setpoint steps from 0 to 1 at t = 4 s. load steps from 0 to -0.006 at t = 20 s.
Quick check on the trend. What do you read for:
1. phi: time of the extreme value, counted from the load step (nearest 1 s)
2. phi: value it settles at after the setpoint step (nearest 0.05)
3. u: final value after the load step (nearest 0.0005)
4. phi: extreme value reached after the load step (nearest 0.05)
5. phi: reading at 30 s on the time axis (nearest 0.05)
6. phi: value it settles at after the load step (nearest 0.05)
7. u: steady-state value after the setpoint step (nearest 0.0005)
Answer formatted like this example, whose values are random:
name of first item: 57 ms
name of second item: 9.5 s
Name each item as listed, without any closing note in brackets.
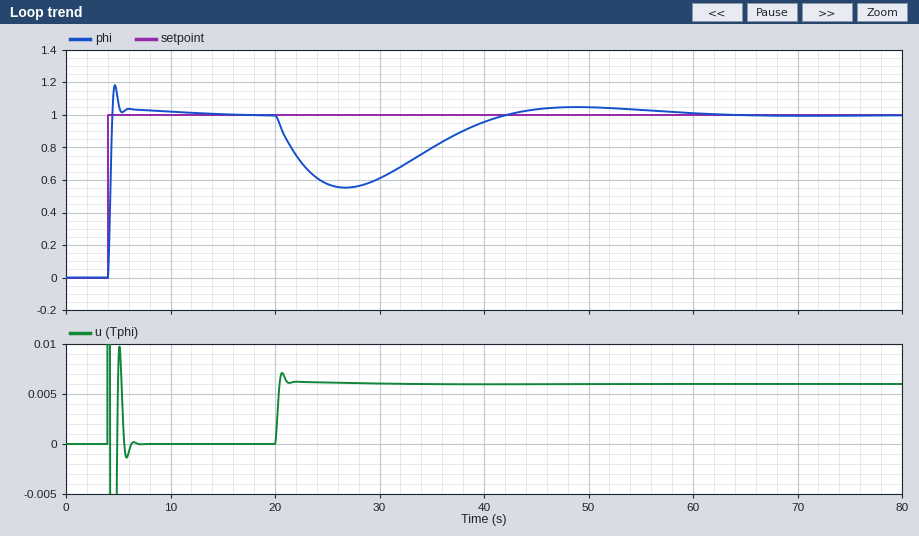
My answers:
phi: time of the extreme value, counted from the load step: 7 s
phi: value it settles at after the setpoint step: 1.00
u: final value after the load step: 0.0060
phi: extreme value reached after the load step: 0.55
phi: reading at 30 s on the time axis: 0.60
phi: value it settles at after the load step: 1.00
u: steady-state value after the setpoint step: 0.0000
